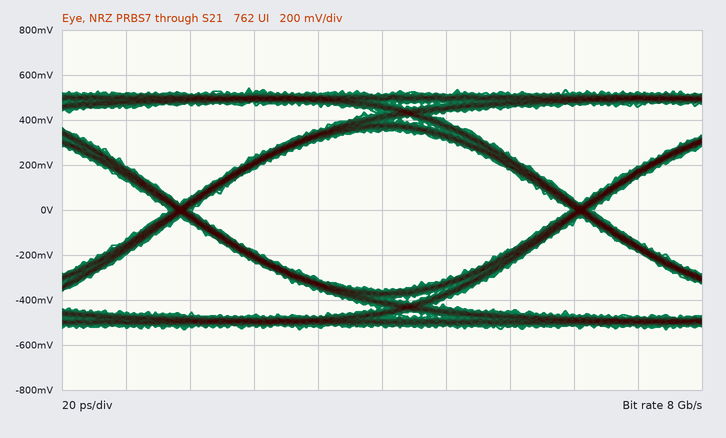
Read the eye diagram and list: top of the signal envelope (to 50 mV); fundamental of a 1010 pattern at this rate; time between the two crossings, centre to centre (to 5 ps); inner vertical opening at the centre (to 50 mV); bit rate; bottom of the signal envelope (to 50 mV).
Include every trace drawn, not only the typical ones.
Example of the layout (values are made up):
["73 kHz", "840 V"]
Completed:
["550 mV", "4 GHz", "125 ps", "700 mV", "8 Gb/s", "-550 mV"]
